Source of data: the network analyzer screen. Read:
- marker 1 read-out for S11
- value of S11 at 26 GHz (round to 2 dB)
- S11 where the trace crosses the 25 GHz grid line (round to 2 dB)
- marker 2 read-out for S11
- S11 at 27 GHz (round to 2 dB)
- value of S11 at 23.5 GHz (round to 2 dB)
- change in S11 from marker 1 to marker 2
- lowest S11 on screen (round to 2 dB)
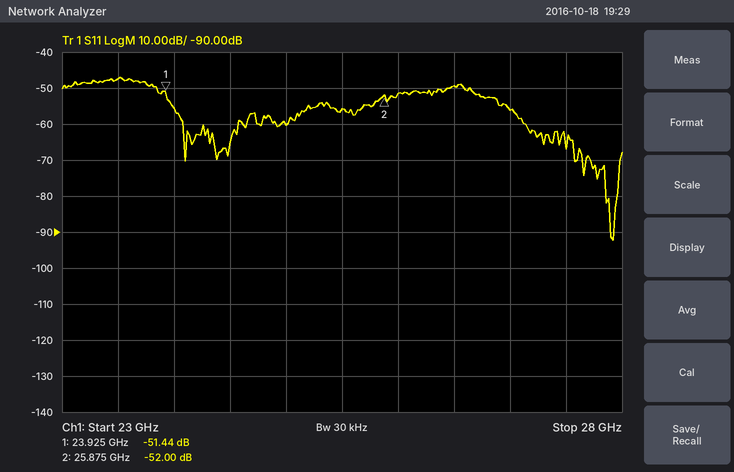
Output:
-51.44 dB
-52 dB
-60 dB
-52.00 dB
-56 dB
-48 dB
-0.56 dB
-92 dB
